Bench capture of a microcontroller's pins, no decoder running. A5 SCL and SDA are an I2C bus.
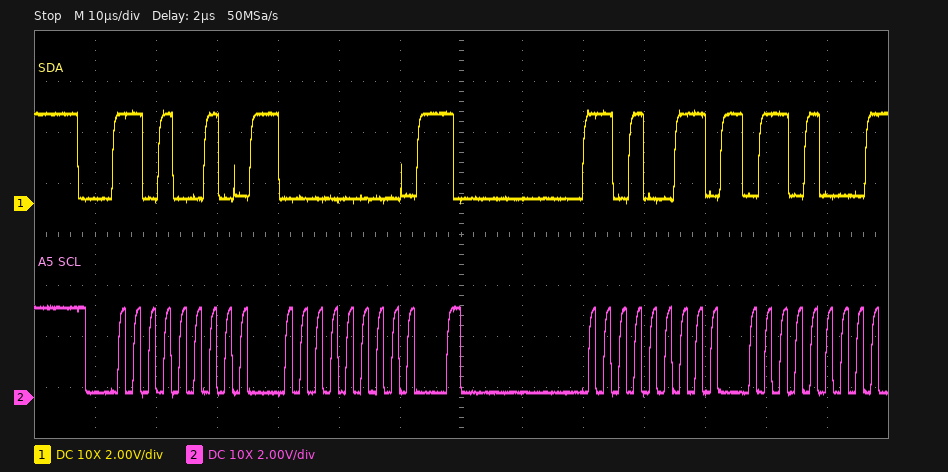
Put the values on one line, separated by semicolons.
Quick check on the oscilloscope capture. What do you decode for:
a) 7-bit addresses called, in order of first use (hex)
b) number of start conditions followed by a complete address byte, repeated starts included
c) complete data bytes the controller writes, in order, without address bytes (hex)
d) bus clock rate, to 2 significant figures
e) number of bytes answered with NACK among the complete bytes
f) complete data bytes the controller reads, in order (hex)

0x69; 2; 00; 400 kHz; 1; 68
